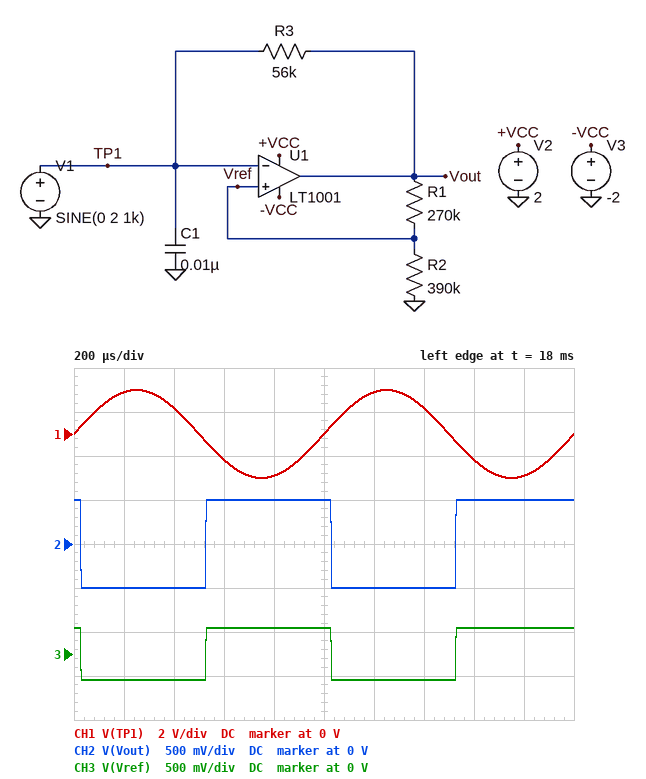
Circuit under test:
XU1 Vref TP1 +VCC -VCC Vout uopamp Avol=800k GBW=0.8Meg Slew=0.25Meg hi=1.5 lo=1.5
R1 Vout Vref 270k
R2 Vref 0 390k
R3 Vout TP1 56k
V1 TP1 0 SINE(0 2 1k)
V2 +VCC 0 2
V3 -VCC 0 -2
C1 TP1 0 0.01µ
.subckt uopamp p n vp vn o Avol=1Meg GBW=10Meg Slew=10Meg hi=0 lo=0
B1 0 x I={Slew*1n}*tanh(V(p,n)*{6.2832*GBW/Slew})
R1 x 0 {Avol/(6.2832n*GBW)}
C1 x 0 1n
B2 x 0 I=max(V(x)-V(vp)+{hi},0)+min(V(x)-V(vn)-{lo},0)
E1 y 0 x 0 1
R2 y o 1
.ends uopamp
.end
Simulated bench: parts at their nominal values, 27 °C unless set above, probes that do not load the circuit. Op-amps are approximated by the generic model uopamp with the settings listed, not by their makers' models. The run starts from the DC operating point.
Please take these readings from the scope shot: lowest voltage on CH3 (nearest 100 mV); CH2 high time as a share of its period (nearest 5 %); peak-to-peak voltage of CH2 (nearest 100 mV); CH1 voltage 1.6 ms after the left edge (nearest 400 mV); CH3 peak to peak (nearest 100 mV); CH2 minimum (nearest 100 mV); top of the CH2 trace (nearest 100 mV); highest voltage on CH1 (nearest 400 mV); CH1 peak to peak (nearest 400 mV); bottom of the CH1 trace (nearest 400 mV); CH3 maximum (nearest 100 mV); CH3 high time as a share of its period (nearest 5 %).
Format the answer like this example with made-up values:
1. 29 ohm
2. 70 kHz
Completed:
1. -300 mV
2. 50 %
3. 1.0 V
4. -1.2 V
5. 600 mV
6. -500 mV
7. 500 mV
8. 2.0 V
9. 4.0 V
10. -2.0 V
11. 300 mV
12. 50 %
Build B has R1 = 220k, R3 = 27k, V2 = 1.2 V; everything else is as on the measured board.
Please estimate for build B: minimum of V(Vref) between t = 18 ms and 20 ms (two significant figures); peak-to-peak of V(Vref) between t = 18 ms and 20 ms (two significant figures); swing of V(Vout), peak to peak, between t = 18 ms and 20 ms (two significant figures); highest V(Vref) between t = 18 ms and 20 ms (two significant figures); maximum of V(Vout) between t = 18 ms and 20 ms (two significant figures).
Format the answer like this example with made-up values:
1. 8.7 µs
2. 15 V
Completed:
1. -320 mV
2. 130 mV
3. 200 mV
4. -190 mV
5. -300 mV
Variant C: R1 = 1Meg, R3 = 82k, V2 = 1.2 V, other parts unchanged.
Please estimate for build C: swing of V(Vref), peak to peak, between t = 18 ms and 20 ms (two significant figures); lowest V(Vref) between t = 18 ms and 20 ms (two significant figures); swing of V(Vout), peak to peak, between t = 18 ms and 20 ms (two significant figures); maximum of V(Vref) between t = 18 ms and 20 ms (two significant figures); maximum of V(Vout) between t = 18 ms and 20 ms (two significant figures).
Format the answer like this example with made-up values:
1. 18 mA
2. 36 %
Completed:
1. 56 mV
2. -140 mV
3. 200 mV
4. -84 mV
5. -300 mV
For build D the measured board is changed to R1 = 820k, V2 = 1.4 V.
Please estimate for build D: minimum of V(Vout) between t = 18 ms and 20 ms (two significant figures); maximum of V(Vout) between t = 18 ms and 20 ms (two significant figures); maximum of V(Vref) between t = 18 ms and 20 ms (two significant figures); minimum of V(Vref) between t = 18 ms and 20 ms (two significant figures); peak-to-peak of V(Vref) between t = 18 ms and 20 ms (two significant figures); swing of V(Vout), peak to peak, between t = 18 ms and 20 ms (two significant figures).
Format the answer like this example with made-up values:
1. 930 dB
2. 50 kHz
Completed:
1. -500 mV
2. -100 mV
3. -32 mV
4. -160 mV
5. 130 mV
6. 400 mV
